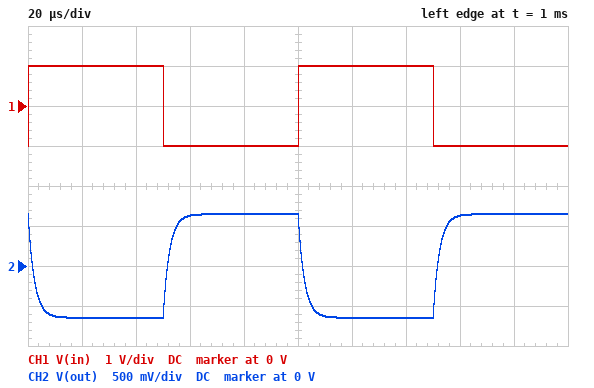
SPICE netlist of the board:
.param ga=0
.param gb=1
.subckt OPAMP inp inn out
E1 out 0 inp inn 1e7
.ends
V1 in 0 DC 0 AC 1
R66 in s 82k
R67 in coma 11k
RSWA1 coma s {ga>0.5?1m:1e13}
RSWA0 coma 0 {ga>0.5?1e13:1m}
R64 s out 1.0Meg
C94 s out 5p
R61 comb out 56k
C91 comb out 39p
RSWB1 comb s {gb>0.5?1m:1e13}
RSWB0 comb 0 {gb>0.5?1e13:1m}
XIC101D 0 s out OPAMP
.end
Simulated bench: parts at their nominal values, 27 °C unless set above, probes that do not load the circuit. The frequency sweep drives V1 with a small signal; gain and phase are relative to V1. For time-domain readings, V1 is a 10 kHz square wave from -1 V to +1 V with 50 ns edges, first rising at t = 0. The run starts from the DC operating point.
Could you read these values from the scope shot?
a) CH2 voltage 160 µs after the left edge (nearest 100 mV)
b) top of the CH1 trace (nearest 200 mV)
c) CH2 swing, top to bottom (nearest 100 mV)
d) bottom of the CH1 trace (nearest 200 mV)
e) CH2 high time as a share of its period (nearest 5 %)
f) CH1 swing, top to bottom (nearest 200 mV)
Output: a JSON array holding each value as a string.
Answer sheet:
["600 mV", "1.0 V", "1.3 V", "-1.0 V", "50 %", "2.0 V"]
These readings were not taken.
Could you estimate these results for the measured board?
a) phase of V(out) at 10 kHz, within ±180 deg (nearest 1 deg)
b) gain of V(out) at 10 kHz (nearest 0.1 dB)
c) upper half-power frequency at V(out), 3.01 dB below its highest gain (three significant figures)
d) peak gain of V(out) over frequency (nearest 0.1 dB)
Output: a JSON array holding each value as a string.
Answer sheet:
["172 deg", "-3.9 dB", "68.2 kHz", "-3.8 dB"]
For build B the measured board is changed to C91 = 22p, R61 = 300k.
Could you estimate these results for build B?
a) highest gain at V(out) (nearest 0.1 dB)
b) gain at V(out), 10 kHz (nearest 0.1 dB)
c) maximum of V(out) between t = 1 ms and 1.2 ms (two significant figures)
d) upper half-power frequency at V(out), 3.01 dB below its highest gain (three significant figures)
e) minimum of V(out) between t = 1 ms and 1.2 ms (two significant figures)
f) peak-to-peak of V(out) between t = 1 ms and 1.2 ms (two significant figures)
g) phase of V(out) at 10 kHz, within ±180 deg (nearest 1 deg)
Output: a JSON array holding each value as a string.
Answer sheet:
["9.0 dB", "8.4 dB", "2.8 V", "25.5 kHz", "-2.8 V", "5.6 V", "159 deg"]
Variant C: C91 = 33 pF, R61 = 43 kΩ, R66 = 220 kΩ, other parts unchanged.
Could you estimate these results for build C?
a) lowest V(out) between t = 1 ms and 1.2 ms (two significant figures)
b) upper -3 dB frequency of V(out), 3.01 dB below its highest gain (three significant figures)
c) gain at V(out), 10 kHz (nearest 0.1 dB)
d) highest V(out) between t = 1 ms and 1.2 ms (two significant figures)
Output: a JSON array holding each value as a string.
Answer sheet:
["-190 mV", "102 kHz", "-14.6 dB", "190 mV"]
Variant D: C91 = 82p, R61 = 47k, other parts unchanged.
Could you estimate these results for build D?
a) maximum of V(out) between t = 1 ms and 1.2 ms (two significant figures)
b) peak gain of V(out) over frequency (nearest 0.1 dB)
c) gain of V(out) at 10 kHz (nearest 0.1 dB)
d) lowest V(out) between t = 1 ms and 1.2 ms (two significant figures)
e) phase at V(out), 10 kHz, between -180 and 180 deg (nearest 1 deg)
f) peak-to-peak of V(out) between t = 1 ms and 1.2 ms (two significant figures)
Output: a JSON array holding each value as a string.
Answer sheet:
["550 mV", "-5.2 dB", "-5.5 dB", "-550 mV", "166 deg", "1.1 V"]
